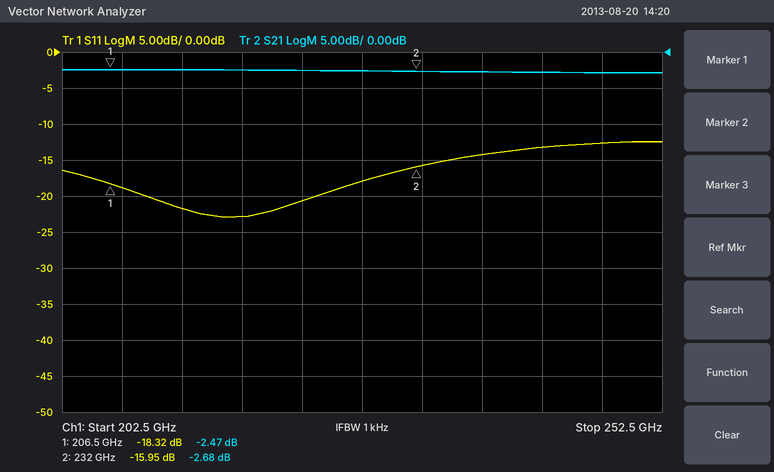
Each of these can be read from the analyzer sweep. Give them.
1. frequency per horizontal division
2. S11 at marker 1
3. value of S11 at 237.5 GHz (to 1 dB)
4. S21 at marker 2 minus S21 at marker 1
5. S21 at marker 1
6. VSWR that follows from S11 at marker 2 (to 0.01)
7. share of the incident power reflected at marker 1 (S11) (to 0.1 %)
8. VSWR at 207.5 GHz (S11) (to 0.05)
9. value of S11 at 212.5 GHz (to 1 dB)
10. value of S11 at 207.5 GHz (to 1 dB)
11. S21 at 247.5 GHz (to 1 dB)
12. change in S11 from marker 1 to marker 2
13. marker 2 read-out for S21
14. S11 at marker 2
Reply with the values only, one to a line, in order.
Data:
5 GHz
-18.32 dB
-14 dB
-0.21 dB
-2.47 dB
1.38
1.5 %
1.25
-22 dB
-19 dB
-3 dB
2.37 dB
-2.68 dB
-15.95 dB
